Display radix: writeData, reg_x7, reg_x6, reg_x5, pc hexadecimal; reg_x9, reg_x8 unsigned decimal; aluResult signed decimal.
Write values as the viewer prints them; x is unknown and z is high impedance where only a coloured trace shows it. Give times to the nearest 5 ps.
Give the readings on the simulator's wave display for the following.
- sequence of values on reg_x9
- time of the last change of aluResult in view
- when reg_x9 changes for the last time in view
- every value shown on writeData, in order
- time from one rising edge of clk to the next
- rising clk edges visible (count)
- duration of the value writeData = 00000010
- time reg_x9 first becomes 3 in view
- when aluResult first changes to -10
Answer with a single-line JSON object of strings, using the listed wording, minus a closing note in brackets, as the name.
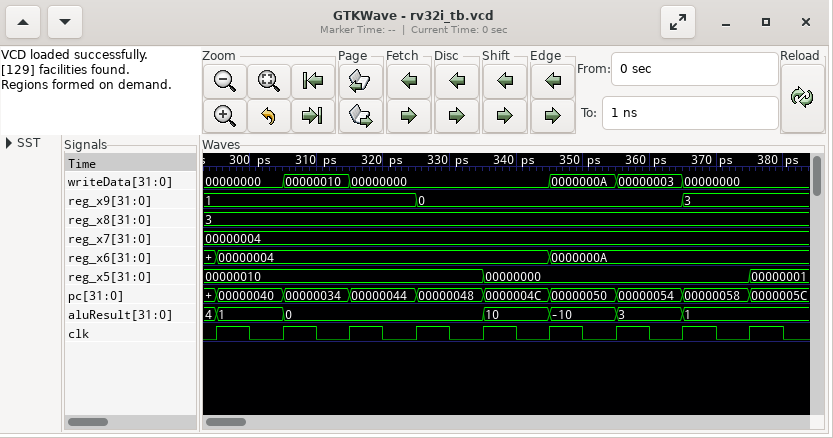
{"sequence of values on reg_x9": "1, 0, 3", "time of the last change of aluResult in view": "365 ps", "when reg_x9 changes for the last time in view": "365 ps", "every value shown on writeData, in order": "00000000, 00000010, 00000000, 0000000A, 00000003, 00000000", "time from one rising edge of clk to the next": "10 ps", "rising clk edges visible": "9", "duration of the value writeData = 00000010": "10 ps", "time reg_x9 first becomes 3 in view": "365 ps", "when aluResult first changes to -10": "345 ps"}
